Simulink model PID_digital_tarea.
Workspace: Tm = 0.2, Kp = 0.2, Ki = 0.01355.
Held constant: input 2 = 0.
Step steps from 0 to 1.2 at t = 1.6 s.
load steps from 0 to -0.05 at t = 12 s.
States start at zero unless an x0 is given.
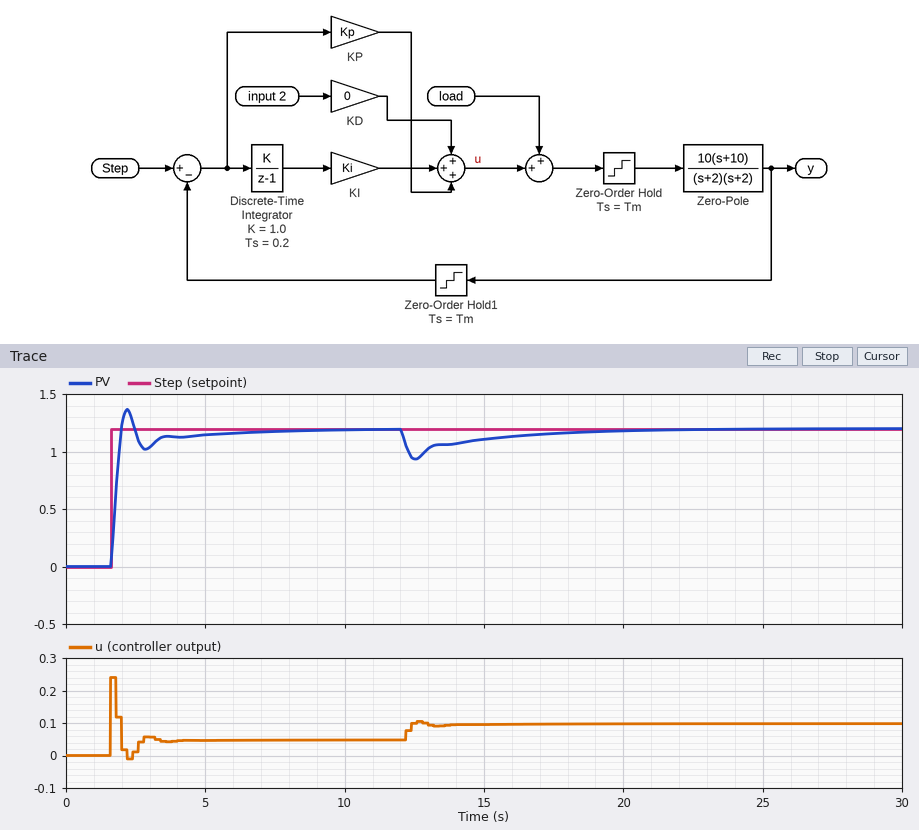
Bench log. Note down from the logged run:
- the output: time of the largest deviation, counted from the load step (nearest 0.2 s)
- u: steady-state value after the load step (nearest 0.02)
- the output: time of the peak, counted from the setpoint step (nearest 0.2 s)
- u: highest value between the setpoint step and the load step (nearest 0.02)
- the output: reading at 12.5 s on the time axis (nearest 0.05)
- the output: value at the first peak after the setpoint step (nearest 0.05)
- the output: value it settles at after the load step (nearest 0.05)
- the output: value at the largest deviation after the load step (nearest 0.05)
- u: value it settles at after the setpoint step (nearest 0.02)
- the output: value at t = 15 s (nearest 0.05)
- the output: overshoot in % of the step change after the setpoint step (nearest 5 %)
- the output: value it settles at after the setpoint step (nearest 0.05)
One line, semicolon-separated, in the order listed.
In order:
0.6 s; 0.10; 0.6 s; 0.24; 0.95; 1.35; 1.20; 0.95; 0.04; 1.10; 15 %; 1.20
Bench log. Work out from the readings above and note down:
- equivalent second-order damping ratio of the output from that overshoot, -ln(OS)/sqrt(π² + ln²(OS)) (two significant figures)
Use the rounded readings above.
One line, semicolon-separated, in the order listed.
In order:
0.52
